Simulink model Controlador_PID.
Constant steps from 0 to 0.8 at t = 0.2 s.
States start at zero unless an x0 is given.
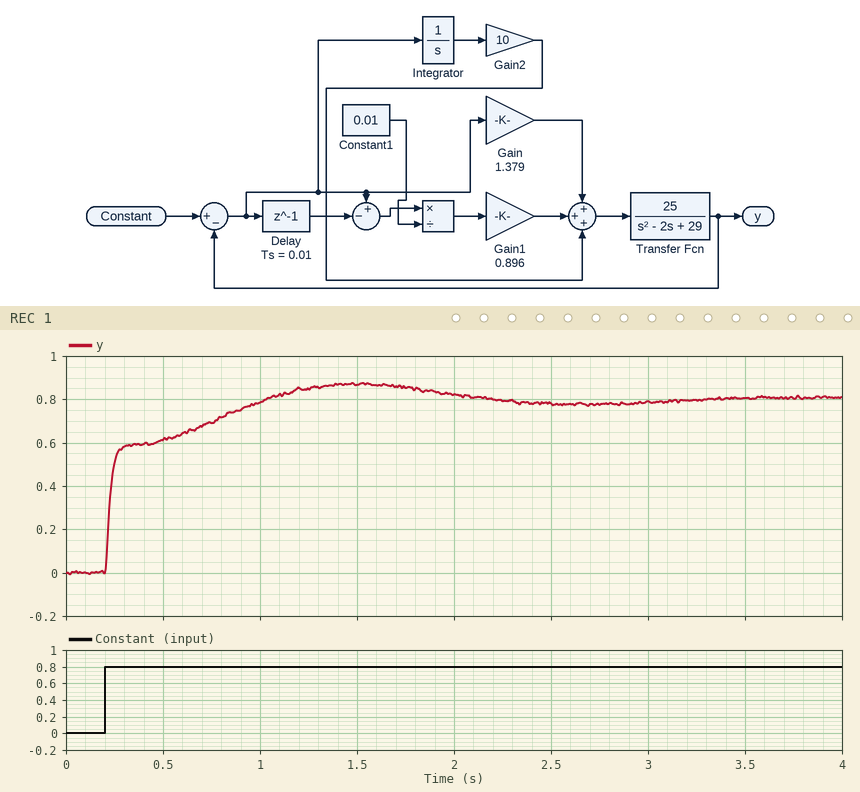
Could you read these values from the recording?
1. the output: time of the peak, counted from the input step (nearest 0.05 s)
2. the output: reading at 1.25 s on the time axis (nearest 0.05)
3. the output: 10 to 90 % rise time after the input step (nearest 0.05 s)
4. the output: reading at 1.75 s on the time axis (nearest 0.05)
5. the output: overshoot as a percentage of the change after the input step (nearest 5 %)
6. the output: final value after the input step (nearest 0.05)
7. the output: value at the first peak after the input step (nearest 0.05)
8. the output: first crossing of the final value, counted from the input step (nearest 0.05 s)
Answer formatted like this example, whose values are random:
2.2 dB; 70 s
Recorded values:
1.30 s; 0.85; 0.60 s; 0.85; 10 %; 0.80; 0.85; 0.85 s
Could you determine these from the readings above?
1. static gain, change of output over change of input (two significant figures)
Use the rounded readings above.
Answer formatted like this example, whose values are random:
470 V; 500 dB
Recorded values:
1.0
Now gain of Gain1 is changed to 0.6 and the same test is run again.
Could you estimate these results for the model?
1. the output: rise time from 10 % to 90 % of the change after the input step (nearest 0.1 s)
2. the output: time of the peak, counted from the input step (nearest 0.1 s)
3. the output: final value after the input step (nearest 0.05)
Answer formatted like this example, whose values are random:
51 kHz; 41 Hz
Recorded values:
0.5 s; 1.1 s; 0.80
